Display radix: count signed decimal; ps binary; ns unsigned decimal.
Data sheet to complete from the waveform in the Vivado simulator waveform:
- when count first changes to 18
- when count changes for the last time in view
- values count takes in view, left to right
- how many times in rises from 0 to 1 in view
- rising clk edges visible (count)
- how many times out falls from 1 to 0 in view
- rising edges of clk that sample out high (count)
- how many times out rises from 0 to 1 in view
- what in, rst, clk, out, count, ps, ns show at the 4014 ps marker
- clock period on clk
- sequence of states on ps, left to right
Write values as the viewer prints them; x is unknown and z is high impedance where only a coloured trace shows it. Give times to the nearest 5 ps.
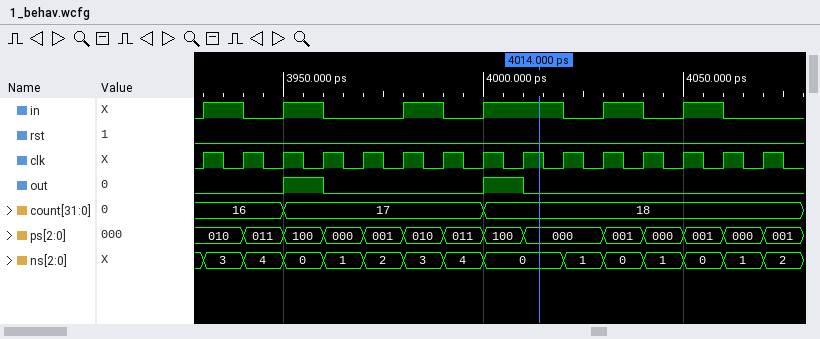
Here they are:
4000 ps
4000 ps
16, 17, 18
6
15
2
2
2
in=1, rst=0, clk=1, out=0, count=18, ps=000, ns=0
10 ps
010, 011, 100, 000, 001, 010, 011, 100, 000, 001, 000, 001, 000, 001
